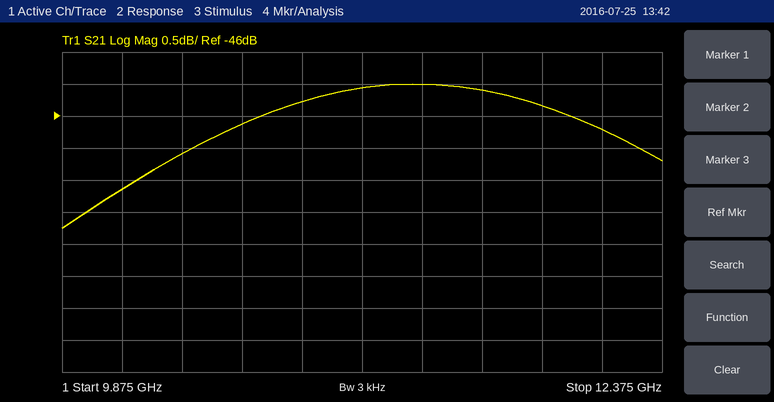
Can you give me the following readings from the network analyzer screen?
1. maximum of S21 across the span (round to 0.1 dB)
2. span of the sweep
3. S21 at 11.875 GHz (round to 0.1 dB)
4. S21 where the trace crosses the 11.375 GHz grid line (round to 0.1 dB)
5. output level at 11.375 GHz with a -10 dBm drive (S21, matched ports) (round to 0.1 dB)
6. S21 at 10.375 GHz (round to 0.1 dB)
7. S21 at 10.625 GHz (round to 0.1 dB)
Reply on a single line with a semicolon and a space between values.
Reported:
-45.5 dB; 2.5 GHz; -45.8 dB; -45.5 dB; -55.5 dBm; -46.6 dB; -46.1 dB
